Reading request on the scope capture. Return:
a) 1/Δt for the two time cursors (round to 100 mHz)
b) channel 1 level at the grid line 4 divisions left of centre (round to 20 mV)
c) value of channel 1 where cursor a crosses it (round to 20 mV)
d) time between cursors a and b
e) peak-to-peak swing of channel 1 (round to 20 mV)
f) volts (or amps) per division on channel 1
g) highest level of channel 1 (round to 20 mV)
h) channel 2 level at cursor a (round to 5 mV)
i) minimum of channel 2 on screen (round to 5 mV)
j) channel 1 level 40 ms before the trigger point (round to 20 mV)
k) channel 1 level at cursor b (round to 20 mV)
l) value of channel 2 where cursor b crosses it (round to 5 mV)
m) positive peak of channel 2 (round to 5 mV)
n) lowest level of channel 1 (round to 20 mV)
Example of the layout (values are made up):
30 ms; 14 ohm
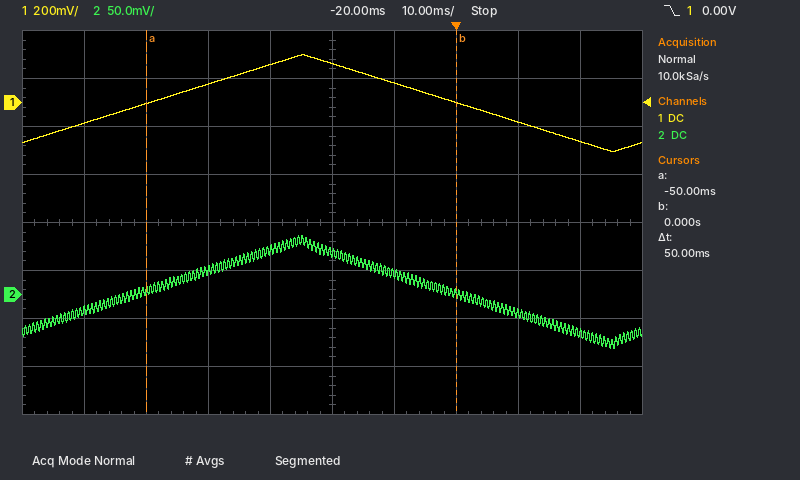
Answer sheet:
20.0 Hz; -80 mV; 0 mV; 50 ms; 400 mV; 200 mV; 200 mV; 5 mV; -55 mV; 80 mV; 0 mV; 0 mV; 60 mV; -200 mV
